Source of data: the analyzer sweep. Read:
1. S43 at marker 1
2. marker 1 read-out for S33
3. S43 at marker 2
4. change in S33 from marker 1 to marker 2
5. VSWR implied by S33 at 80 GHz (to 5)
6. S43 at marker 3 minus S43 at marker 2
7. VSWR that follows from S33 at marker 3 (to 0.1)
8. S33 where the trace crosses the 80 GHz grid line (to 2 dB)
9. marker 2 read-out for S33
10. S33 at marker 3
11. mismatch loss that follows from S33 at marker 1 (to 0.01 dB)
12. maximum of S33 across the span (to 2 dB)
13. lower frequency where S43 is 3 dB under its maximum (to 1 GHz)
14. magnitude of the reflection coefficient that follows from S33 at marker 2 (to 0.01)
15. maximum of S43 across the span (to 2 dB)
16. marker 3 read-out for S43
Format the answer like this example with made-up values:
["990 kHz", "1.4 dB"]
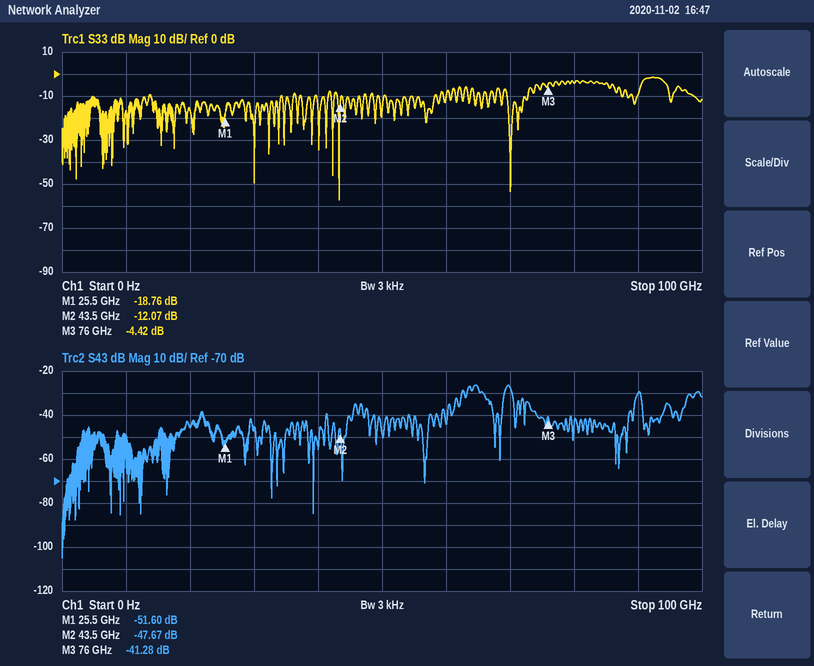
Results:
["-51.60 dB", "-18.76 dB", "-47.67 dB", "6.69 dB", "5", "6.39 dB", "4.0", "-4 dB", "-12.07 dB", "-4.42 dB", "0.06 dB", "-2 dB", "63 GHz", "0.25", "-26 dB", "-41.28 dB"]
